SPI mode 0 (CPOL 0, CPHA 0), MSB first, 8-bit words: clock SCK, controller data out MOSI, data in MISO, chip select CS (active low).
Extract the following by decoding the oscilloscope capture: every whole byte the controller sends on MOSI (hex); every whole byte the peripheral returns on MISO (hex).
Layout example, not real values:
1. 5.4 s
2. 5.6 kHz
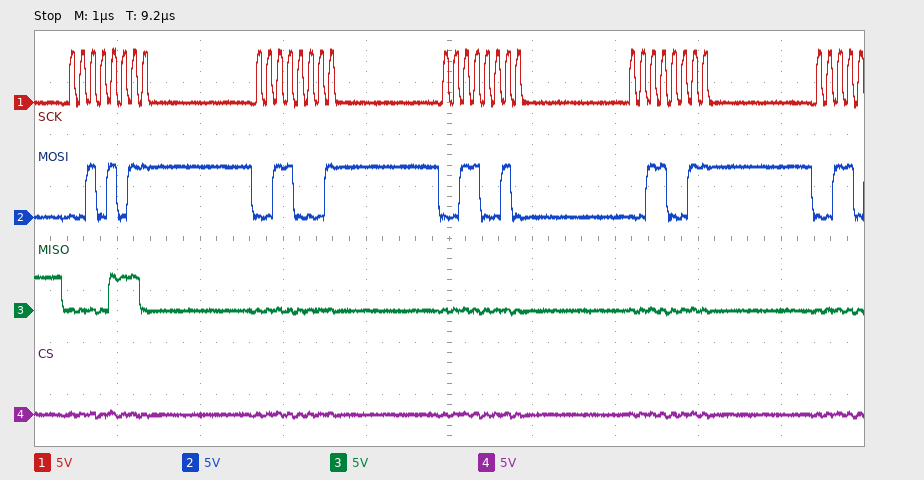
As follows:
1. 2B 31 32 33
2. 0E 00 00 00
